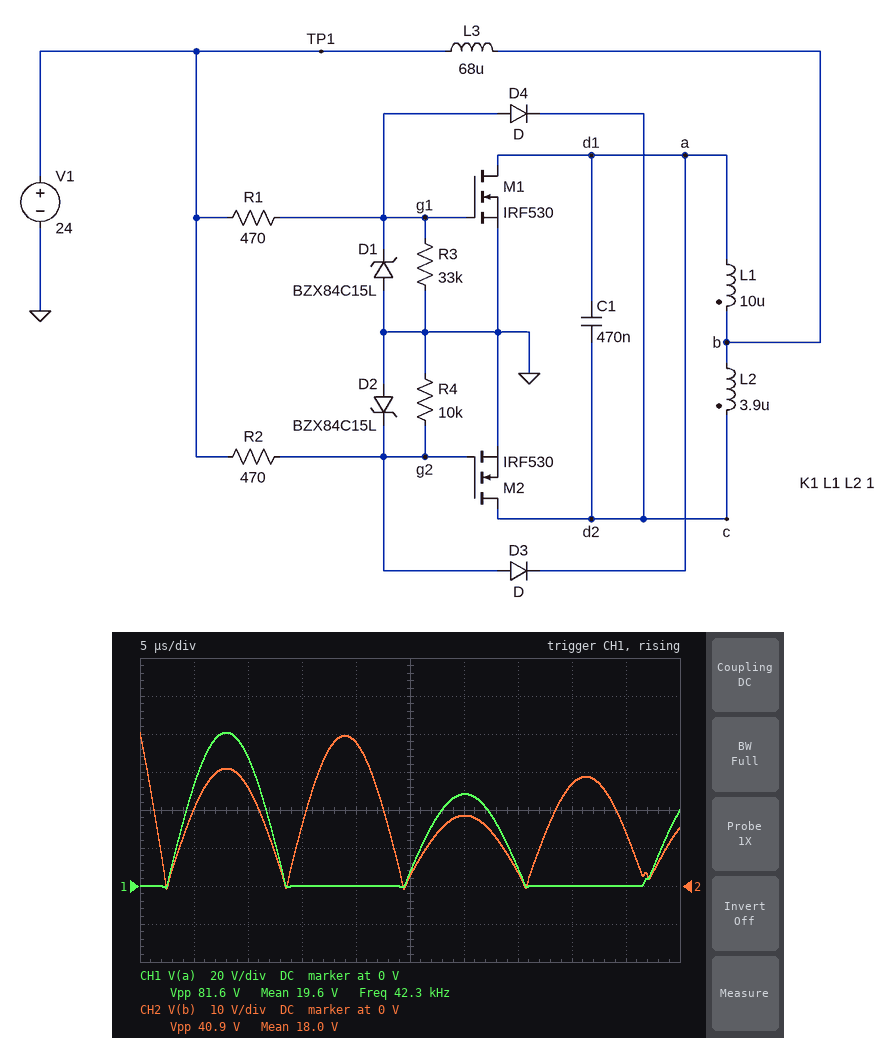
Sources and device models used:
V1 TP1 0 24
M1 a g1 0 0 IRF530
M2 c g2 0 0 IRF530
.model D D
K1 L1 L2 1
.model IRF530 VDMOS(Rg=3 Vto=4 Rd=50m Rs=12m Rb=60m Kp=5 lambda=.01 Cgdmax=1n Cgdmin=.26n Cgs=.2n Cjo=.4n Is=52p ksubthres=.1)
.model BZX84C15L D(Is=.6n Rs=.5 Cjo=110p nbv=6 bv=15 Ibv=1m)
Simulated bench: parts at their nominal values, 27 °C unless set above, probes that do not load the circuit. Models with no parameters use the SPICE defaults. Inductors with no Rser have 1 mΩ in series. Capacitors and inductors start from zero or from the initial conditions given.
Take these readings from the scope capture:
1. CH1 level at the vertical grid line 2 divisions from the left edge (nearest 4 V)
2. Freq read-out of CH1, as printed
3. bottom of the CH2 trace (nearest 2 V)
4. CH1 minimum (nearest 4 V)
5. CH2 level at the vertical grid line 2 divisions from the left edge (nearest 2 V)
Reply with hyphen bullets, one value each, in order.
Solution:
- 68 V
- 42.3 kHz
- 0 V
- 0 V
- 26 V
